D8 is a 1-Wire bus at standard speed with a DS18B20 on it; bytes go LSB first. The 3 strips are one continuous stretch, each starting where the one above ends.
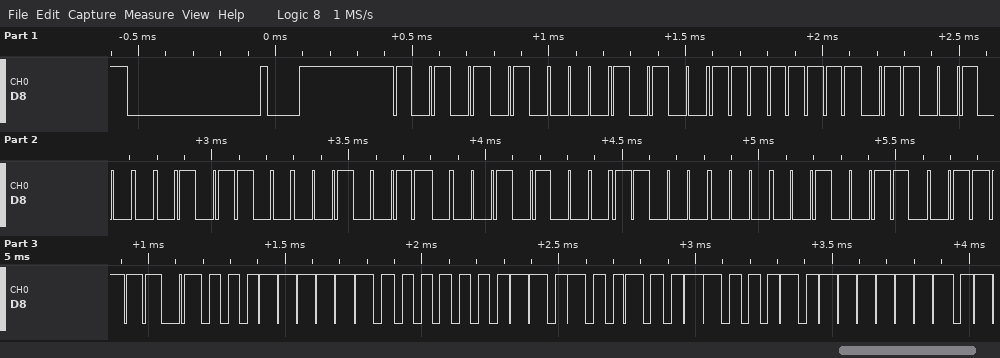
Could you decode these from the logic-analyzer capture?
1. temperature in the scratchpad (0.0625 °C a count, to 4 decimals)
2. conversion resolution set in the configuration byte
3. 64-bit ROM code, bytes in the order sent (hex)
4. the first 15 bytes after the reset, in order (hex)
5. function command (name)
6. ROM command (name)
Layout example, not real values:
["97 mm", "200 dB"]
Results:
["31.5000 °C", "12 bits", "28 FF 26 34 64 14 03 64", "55 28 FF 26 34 64 14 03 64 BE F8 01 4B 46 7F", "Read Scratchpad", "Match ROM"]
